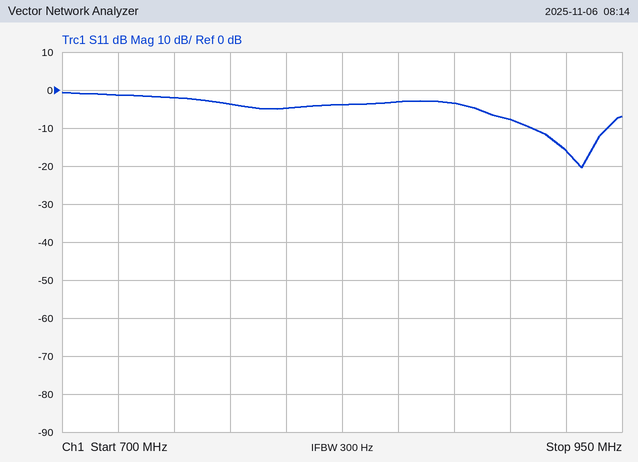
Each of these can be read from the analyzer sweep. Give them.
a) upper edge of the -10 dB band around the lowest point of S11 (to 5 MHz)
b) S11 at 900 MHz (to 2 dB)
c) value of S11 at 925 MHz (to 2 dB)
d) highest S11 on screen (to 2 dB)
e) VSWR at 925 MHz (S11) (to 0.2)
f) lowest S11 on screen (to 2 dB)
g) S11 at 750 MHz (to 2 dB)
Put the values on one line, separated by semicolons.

945 MHz; -8 dB; -16 dB; 0 dB; 1.4; -20 dB; -2 dB
